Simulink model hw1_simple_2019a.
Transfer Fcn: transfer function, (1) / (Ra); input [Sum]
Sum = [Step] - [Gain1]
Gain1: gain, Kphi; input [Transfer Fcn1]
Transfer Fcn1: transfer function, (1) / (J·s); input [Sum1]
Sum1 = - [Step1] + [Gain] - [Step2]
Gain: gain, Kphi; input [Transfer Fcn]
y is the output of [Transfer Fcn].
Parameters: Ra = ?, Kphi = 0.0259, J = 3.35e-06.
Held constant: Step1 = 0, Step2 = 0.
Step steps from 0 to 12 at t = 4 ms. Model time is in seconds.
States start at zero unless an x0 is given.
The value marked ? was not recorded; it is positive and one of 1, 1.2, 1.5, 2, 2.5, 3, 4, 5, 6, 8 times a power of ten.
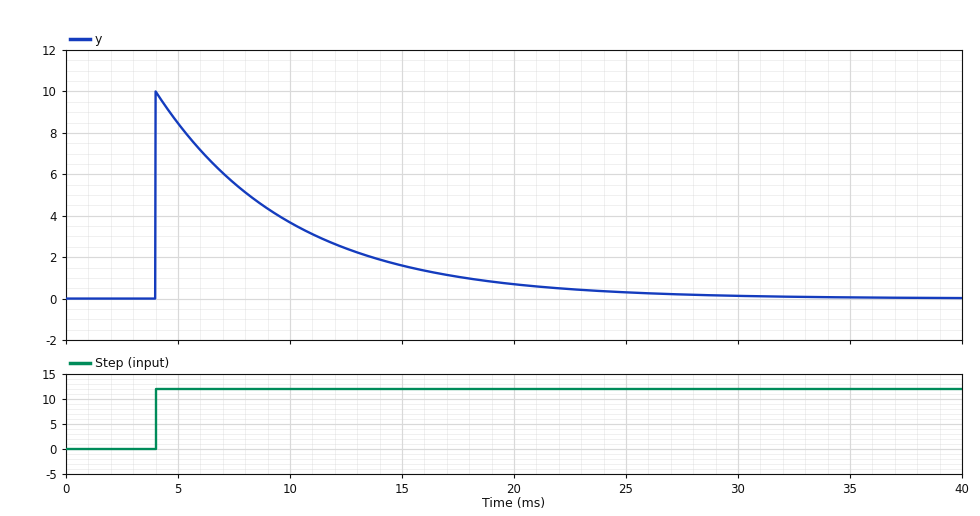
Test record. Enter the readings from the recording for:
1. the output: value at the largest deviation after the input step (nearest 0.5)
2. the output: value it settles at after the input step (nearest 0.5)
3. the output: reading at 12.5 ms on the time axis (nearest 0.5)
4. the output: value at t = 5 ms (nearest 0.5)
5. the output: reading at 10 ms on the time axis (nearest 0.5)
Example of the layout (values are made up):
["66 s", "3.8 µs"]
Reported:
["10.0", "0.0", "2.5", "8.5", "3.5"]
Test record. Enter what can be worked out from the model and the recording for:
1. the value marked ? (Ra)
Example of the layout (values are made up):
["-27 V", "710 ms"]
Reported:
["1.2"]
